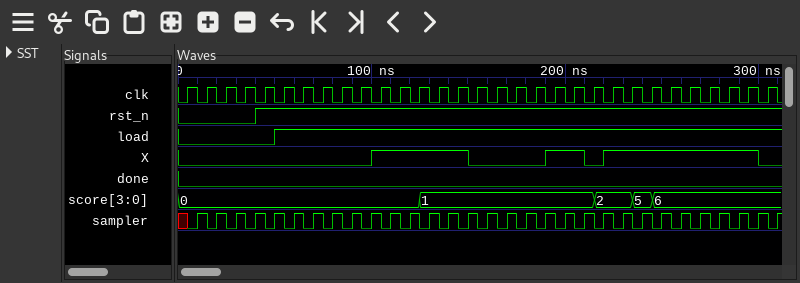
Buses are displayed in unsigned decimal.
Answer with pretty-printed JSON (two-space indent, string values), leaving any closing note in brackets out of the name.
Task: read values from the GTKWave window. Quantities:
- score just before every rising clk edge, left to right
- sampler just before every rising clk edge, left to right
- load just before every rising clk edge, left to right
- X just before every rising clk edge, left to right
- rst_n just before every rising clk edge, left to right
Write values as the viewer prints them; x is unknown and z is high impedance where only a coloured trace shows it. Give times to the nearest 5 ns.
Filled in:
{
  "score just before every rising clk edge, left to right": "0, 0, 0, 0, 0, 0, 0, 0, 0, 0, 0, 0, 0, 1, 1, 1, 1, 1, 1, 1, 1, 1, 2, 2, 5, 6, 6, 6, 6, 6, 6",
  "sampler just before every rising clk edge, left to right": "x 1 1 1 1 1 1 1 1 1 1 1 1 1 1 1 1 1 1 1 1 1 1 1 1 1 1 1 1 1 1",
  "load just before every rising clk edge, left to right": "0 0 0 0 0 1 1 1 1 1 1 1 1 1 1 1 1 1 1 1 1 1 1 1 1 1 1 1 1 1 1",
  "X just before every rising clk edge, left to right": "0 0 0 0 0 0 0 0 0 0 1 1 1 1 1 0 0 0 0 1 1 0 1 1 1 1 1 1 1 1 0",
  "rst_n just before every rising clk edge, left to right": "0 0 0 0 1 1 1 1 1 1 1 1 1 1 1 1 1 1 1 1 1 1 1 1 1 1 1 1 1 1 1"
}
